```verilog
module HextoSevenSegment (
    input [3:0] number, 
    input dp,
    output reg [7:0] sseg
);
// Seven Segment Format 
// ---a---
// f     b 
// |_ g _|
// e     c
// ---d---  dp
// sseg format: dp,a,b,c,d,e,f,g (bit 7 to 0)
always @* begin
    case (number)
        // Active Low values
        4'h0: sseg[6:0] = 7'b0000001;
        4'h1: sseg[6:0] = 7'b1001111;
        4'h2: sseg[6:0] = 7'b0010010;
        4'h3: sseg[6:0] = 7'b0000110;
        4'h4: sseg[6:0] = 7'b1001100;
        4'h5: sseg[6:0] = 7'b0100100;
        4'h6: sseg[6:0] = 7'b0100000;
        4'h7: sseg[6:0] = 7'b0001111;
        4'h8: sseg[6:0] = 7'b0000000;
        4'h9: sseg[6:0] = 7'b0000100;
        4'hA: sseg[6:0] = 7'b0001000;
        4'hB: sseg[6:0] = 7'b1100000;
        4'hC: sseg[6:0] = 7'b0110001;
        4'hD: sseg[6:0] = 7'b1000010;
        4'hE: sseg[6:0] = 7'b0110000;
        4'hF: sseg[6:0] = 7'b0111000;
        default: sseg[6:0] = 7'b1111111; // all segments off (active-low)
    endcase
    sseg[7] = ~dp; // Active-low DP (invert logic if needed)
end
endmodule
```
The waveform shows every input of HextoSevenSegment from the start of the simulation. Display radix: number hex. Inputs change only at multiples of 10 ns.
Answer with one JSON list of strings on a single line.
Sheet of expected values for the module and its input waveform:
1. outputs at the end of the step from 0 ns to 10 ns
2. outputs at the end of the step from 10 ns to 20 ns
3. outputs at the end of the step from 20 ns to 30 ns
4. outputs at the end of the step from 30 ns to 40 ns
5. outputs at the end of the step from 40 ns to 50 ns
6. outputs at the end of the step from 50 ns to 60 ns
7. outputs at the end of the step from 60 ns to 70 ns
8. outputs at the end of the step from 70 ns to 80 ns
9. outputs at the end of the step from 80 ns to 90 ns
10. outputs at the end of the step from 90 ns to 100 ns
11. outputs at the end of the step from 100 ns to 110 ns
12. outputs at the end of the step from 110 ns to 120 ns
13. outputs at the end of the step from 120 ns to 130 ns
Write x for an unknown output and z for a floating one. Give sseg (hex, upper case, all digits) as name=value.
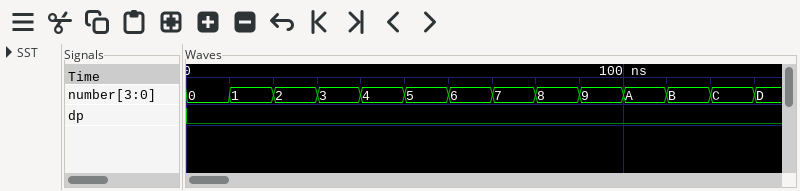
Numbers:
["sseg=81", "sseg=CF", "sseg=92", "sseg=86", "sseg=CC", "sseg=A4", "sseg=A0", "sseg=8F", "sseg=80", "sseg=84", "sseg=88", "sseg=E0", "sseg=B1"]
